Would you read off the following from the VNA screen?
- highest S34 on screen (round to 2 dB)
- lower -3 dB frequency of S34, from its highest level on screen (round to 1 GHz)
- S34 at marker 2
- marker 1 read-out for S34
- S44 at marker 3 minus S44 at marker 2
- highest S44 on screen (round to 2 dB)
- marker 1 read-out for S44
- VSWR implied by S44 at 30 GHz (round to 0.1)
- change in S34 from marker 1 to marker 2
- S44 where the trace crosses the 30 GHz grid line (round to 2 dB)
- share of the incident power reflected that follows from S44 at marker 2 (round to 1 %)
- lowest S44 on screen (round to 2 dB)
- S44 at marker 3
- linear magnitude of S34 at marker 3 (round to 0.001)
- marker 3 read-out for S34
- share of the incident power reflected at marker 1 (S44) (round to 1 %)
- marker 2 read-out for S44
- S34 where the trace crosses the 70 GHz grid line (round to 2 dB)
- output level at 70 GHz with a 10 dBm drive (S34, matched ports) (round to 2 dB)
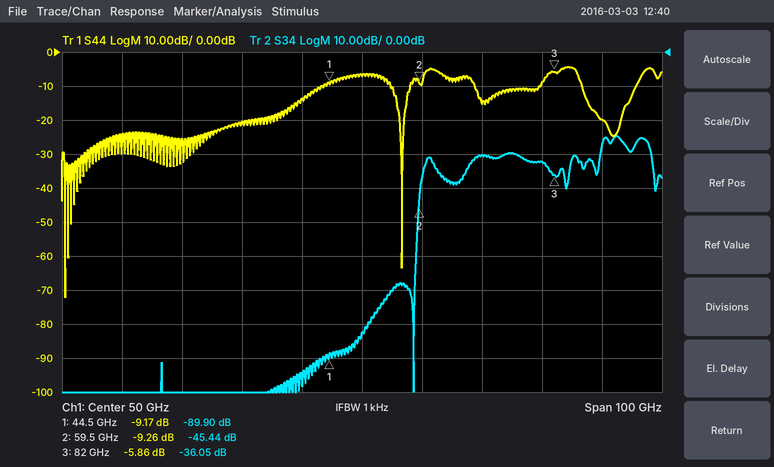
-24 dB
90 GHz
-45.44 dB
-89.90 dB
3.40 dB
-4 dB
-9.17 dB
1.2
44.46 dB
-20 dB
12 %
-72 dB
-5.86 dB
0.016
-36.05 dB
12 %
-9.26 dB
-30 dB
-20 dBm
